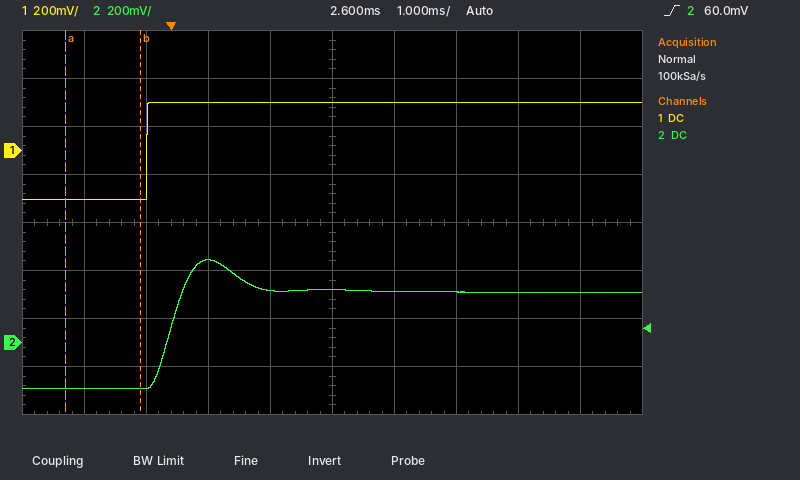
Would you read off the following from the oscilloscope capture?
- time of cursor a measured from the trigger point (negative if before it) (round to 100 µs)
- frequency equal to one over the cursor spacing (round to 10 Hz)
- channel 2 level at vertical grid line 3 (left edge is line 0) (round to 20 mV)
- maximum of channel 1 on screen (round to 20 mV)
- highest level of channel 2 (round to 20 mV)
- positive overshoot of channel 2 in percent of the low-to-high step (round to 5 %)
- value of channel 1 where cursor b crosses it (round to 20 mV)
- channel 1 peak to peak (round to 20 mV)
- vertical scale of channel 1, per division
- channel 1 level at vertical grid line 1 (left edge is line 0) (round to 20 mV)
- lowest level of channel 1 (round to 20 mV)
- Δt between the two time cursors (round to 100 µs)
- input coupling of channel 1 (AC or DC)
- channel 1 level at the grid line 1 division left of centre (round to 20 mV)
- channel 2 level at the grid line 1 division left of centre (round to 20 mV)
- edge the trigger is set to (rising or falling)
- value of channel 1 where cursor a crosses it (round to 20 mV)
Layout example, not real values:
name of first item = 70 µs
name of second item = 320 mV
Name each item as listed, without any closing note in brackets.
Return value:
time of cursor a measured from the trigger point (negative if before it) = -1.7 ms
frequency equal to one over the cursor spacing = 830 Hz
channel 2 level at vertical grid line 3 (left edge is line 0) = 340 mV
maximum of channel 1 on screen = 200 mV
highest level of channel 2 = 340 mV
positive overshoot of channel 2 in percent of the low-to-high step = 35 %
value of channel 1 where cursor b crosses it = -200 mV
channel 1 peak to peak = 400 mV
vertical scale of channel 1, per division = 200 mV
channel 1 level at vertical grid line 1 (left edge is line 0) = -200 mV
lowest level of channel 1 = -200 mV
Δt between the two time cursors = 1.2 ms
input coupling of channel 1 = DC
channel 1 level at the grid line 1 division left of centre = 200 mV
channel 2 level at the grid line 1 division left of centre = 220 mV
edge the trigger is set to = rising
value of channel 1 where cursor a crosses it = -200 mV
